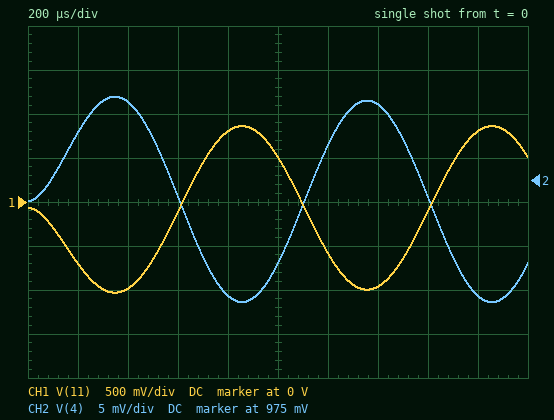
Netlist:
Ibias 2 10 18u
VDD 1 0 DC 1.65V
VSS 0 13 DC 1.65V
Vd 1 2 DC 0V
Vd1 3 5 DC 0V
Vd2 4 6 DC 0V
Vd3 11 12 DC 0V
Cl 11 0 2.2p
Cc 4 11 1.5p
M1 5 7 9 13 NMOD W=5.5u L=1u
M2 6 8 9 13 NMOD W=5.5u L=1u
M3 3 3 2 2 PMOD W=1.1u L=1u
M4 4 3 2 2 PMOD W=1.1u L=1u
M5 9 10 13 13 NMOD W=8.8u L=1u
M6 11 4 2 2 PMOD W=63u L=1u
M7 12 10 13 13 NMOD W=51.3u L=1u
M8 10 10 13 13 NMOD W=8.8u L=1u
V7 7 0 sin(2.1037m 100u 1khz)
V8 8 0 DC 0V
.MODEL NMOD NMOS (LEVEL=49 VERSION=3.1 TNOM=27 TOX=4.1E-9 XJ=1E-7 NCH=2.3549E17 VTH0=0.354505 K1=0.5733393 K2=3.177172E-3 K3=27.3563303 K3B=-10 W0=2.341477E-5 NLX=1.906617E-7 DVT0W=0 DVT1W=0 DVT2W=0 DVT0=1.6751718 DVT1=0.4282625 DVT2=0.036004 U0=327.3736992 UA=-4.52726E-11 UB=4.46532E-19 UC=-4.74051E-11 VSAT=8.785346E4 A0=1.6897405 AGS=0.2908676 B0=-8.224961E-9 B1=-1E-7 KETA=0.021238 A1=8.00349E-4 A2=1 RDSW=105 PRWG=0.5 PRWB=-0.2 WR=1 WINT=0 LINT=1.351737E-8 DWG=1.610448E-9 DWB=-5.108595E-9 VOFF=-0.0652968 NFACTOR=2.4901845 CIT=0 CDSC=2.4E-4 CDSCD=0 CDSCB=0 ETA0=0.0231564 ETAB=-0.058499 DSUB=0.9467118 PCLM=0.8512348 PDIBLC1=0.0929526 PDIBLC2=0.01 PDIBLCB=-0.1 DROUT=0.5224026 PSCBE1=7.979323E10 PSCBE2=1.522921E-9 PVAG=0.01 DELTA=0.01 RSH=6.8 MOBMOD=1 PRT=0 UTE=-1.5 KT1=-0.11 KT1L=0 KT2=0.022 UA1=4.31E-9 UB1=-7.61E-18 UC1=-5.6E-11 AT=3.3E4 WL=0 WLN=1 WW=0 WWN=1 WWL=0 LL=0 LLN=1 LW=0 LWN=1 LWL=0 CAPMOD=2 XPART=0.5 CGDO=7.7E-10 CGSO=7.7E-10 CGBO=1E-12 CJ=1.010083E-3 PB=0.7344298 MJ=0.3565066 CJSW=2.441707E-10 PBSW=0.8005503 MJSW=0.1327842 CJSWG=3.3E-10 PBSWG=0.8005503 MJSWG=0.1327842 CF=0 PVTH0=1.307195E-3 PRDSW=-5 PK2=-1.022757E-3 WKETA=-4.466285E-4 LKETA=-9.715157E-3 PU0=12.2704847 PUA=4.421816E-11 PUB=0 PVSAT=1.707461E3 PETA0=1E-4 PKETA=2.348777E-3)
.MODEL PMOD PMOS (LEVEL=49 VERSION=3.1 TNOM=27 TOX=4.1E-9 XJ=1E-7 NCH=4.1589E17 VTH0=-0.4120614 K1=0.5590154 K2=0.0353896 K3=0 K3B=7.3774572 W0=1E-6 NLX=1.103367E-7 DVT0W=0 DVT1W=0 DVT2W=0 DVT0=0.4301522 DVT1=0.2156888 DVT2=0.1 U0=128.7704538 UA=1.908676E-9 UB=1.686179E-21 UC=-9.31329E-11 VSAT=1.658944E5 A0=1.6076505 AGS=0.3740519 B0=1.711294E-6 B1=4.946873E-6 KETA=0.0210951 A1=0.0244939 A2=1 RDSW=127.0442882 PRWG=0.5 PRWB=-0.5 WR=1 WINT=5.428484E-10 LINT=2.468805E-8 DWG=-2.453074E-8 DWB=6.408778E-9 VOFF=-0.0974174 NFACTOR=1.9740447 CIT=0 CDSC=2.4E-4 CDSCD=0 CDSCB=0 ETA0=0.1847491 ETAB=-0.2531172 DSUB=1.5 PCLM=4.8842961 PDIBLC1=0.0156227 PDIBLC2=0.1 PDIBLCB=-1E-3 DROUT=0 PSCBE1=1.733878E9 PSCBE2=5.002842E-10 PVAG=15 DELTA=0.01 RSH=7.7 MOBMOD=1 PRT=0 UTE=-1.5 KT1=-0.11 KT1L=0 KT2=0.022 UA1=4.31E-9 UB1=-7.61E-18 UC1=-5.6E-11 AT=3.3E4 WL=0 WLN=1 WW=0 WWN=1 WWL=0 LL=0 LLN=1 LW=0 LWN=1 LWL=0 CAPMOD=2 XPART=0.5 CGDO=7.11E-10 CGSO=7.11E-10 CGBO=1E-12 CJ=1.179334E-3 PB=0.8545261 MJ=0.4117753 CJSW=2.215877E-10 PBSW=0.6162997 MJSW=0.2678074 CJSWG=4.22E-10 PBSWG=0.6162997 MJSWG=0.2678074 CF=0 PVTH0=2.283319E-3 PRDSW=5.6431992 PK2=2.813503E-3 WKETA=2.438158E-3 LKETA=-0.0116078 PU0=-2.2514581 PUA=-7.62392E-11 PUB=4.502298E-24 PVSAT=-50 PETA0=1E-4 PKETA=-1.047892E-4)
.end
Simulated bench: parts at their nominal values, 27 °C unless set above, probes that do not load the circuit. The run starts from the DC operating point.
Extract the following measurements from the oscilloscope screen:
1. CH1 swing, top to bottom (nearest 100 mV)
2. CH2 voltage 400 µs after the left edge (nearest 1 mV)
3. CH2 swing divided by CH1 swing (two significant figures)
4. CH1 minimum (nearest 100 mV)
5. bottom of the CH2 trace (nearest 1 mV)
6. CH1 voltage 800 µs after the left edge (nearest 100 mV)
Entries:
1.9 V
984 mV
0.012
-1.0 V
961 mV
800 mV
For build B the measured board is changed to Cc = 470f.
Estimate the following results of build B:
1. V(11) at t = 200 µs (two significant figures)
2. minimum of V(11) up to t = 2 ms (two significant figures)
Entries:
-1.0 V
-1.2 V
